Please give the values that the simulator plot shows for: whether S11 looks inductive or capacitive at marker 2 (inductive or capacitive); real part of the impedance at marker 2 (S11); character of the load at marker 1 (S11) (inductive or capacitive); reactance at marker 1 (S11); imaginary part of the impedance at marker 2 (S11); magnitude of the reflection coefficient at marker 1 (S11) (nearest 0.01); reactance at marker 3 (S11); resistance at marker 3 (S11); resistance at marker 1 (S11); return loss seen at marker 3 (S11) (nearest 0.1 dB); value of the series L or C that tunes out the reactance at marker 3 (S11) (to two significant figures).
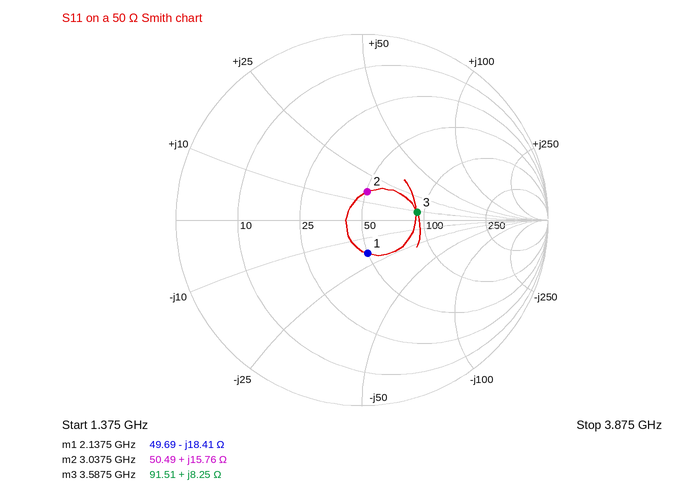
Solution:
inductive
50.49 Ω
capacitive
-18.41 Ω
+15.76 Ω
0.18
+8.25 Ω
91.51 Ω
49.69 Ω
10.5 dB
5.4 pF
